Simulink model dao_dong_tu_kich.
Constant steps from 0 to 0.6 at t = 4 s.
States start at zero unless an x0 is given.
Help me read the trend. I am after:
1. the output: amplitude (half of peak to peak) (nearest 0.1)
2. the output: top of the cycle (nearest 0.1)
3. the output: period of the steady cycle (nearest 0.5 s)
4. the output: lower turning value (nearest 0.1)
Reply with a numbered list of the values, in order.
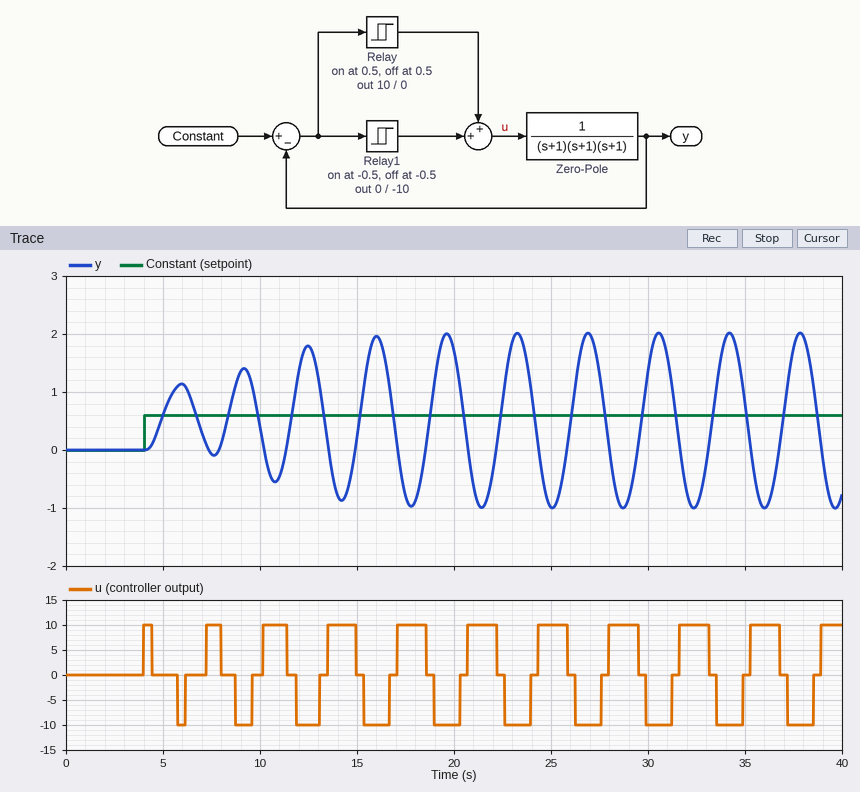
1. 1.5
2. 2.0
3. 3.5 s
4. -1.0
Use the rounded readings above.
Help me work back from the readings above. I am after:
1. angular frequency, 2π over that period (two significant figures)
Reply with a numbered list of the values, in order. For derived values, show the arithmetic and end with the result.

1. 2π / 3.5 = 1.8 rad/s
